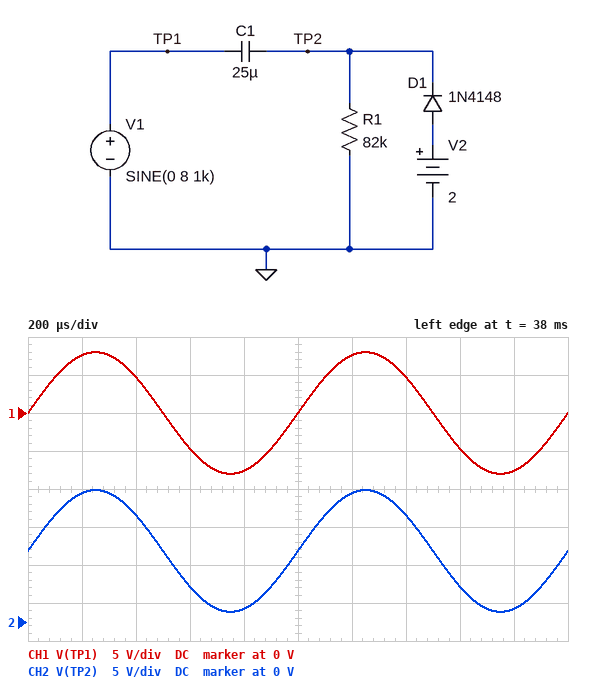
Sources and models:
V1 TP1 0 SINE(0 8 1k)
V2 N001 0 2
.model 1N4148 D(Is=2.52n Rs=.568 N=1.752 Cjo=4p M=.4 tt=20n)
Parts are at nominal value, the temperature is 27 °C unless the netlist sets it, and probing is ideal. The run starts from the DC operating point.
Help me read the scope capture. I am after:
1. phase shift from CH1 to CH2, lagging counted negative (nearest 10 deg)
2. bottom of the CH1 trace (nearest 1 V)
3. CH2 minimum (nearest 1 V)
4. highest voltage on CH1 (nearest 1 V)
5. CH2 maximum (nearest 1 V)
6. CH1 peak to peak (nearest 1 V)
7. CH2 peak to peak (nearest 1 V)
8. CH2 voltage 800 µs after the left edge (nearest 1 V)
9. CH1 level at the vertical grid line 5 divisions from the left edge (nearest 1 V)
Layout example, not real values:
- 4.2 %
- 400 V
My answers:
- 0 deg
- -8 V
- 1 V
- 8 V
- 17 V
- 16 V
- 16 V
- 2 V
- 0 V
